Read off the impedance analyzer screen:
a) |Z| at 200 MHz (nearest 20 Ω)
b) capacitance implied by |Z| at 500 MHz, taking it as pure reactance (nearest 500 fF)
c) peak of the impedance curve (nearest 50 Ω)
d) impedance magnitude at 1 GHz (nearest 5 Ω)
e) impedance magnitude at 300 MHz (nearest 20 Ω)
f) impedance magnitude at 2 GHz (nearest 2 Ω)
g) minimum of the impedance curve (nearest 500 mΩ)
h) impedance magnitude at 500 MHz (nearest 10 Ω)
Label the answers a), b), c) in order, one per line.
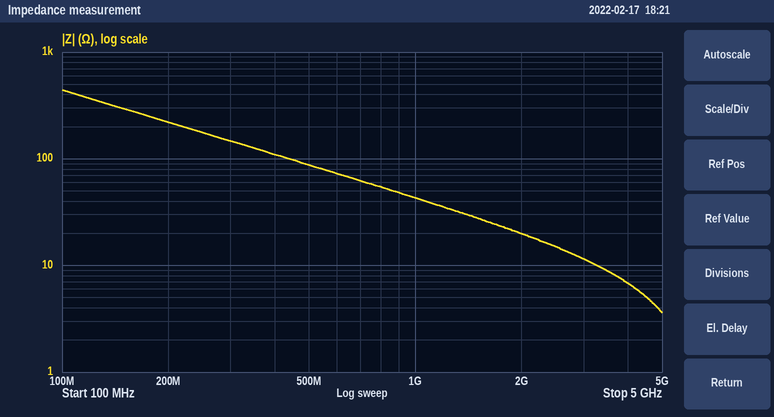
a) 220 Ω
b) 3.5 pF
c) 450 Ω
d) 45 Ω
e) 140 Ω
f) 20 Ω
g) 3.5 Ω
h) 90 Ω
